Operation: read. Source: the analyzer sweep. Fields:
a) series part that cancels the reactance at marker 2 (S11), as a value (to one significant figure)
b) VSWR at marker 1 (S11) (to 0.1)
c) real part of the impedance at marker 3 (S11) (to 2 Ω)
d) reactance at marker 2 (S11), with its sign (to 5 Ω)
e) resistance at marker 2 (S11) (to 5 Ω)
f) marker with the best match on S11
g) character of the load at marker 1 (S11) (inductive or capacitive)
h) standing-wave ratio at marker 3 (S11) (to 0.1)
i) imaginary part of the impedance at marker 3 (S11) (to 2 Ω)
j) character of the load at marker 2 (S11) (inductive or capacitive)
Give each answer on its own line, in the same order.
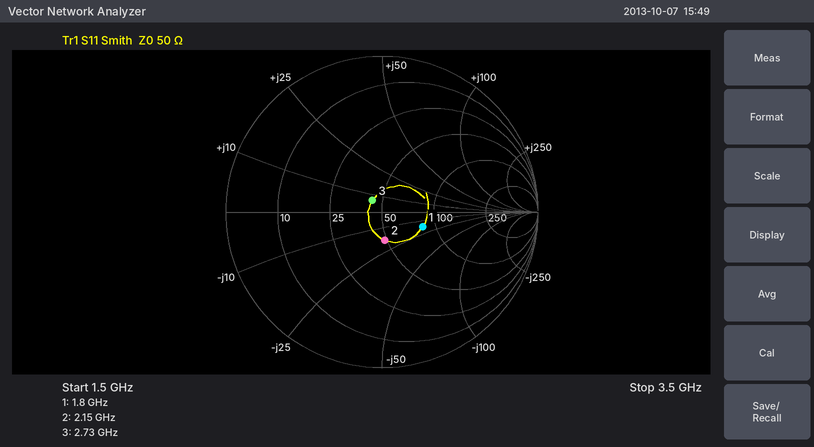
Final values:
1 nH
1.8
44 Ω
-20 Ω
50 Ω
marker 3
capacitive
1.2
+6 Ω
capacitive
